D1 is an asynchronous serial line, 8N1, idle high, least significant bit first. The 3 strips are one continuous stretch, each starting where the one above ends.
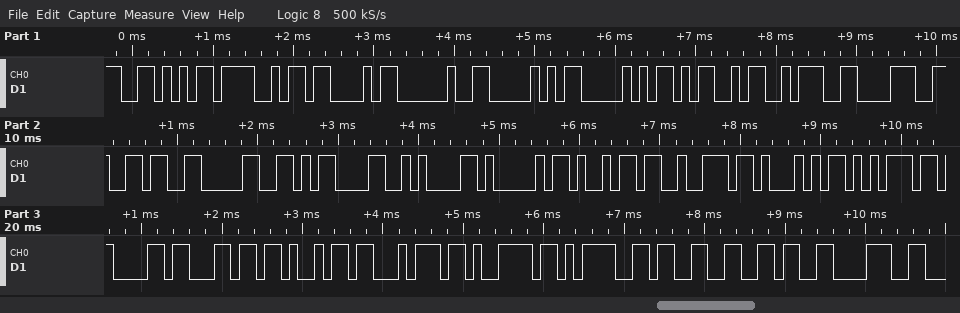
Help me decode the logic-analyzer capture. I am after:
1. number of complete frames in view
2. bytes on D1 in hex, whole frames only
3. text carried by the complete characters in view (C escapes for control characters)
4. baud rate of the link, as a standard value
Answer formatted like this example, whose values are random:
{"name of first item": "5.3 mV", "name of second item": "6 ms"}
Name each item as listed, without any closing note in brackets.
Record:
{"number of complete frames in view": "27", "bytes on D1 in hex, whole frames only": "0x56 0x4F 0x43 0x20 0x50 0x50 0x4D 0x3A 0x38 0x36 0x30 0x0D 0x0A 0x41 0x69 0x72 0x51 0x75 0x61 0x6C 0x69 0x74 0x79 0x3D 0x33 0x36 0x38", "text carried by the complete characters in view": "\"VOC PPM:860\\r\\nAirQuality=368\"", "baud rate of the link, as a standard value": "9600 baud"}
